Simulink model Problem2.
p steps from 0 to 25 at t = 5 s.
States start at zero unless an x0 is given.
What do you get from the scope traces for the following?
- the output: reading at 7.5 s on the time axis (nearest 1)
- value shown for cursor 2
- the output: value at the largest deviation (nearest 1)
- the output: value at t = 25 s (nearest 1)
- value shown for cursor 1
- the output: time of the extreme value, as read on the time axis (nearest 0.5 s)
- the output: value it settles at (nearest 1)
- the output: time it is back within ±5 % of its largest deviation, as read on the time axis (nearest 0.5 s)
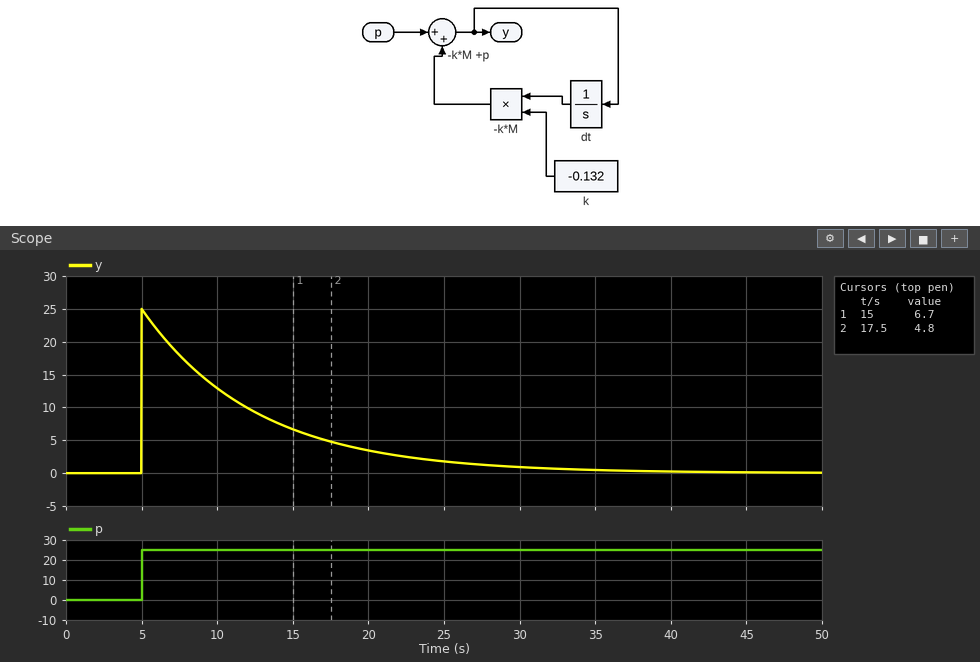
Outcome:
18
4.8
25
2
6.7
5.0 s
0
27.5 s
